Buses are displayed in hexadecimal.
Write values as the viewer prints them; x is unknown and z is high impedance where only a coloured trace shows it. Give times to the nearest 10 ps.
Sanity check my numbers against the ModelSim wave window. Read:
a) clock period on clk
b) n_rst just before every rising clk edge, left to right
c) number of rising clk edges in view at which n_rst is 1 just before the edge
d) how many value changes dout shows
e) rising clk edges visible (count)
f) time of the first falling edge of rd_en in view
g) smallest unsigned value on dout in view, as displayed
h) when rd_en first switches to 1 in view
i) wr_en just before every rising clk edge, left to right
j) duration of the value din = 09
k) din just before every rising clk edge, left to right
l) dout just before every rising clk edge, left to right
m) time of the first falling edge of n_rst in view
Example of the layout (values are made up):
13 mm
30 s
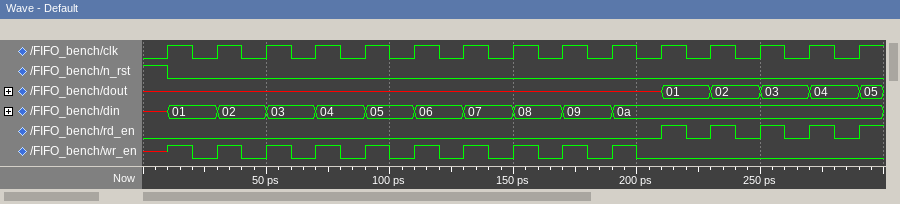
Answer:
20 ps
1 0 0 0 0 0 0 0 0 0 0 0 0 0 0
1
5
15
220 ps
01
210 ps
x 0 0 0 0 0 0 0 0 0 0 0 0 0 0
20 ps
x, 01, 02, 03, 04, 05, 06, 07, 08, 09, 0a, 0a, 0a, 0a, 0a
x, x, x, x, x, x, x, x, x, x, x, 01, 02, 03, 04
10 ps
